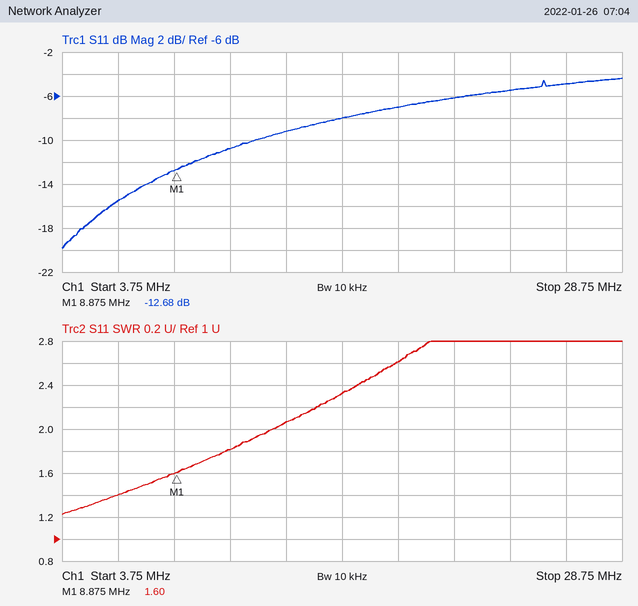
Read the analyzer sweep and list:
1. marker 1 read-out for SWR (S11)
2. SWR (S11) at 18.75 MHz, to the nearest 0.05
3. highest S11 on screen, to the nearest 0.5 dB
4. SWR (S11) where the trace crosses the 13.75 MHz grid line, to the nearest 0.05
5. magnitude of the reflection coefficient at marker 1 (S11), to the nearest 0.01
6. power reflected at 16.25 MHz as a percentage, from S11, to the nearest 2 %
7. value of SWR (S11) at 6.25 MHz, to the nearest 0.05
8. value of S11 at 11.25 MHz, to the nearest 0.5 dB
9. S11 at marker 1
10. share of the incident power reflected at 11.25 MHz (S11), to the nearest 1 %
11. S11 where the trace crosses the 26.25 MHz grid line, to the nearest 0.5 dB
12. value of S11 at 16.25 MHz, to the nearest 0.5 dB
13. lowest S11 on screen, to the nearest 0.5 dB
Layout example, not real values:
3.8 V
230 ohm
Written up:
1.60
2.60
-4.5 dB
2.05
0.23
16 %
1.40
-11.0 dB
-12.68 dB
8 %
-5.0 dB
-8.0 dB
-20.0 dB
